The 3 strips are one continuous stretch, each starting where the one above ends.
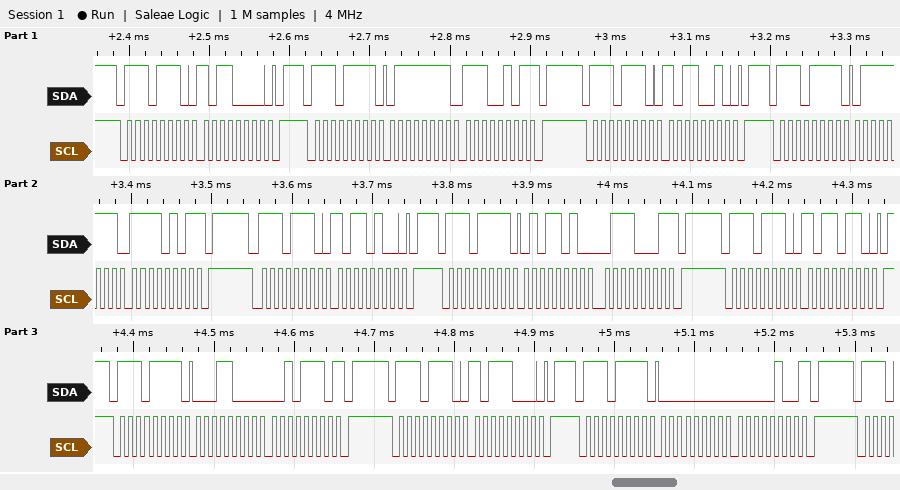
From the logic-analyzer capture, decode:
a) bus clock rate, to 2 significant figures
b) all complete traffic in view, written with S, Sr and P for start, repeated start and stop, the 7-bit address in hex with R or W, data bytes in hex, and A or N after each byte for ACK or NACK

100 kHz
S 77W A B0 A P S 77R A 7F A E5 N P S 77W A B2 A P S 77R A 7F A F5 N P S 77W A B4 A P S 77R A 5A A 71 N P S 77W A B6 A P S 77R A 18 A 2E N P S 77W A B8 A P S 77R A 00 A 04 N P
